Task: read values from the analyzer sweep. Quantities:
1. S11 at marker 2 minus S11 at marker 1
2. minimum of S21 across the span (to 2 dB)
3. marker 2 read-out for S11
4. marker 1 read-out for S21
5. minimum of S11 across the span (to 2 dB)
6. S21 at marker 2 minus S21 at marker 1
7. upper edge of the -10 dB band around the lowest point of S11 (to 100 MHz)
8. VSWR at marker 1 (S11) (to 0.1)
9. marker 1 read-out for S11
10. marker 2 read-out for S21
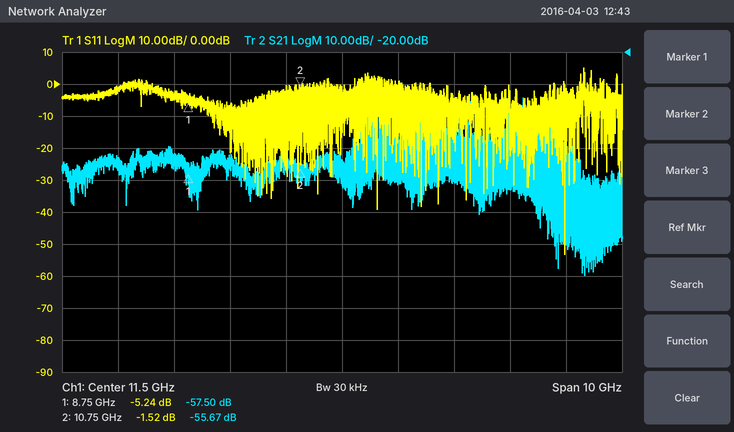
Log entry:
3.72 dB
-90 dB
-1.52 dB
-57.50 dB
-54 dB
1.83 dB
15.5 GHz
3.4
-5.24 dB
-55.67 dB
